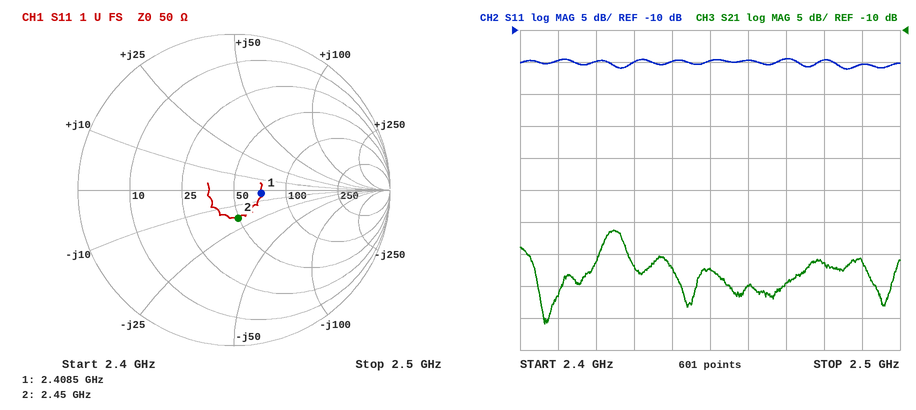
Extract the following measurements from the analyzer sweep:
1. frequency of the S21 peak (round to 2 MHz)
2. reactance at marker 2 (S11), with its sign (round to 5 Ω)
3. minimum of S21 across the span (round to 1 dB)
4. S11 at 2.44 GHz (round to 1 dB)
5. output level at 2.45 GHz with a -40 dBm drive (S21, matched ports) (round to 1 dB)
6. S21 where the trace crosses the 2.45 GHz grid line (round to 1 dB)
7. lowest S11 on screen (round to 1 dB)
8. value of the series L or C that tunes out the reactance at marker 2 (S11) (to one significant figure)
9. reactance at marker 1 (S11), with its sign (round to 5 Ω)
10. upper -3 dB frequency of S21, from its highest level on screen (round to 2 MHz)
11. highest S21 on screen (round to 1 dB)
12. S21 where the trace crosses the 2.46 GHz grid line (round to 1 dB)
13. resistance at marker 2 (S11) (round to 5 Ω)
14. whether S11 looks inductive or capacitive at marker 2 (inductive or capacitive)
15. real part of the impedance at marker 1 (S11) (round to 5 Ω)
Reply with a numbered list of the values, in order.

1. 2.424 GHz
2. -20 Ω
3. -56 dB
4. -15 dB
5. -87 dBm
6. -47 dB
7. -16 dB
8. 1 nH
9. -5 Ω
10. 2.428 GHz
11. -41 dB
12. -50 dB
13. 50 Ω
14. capacitive
15. 70 Ω
